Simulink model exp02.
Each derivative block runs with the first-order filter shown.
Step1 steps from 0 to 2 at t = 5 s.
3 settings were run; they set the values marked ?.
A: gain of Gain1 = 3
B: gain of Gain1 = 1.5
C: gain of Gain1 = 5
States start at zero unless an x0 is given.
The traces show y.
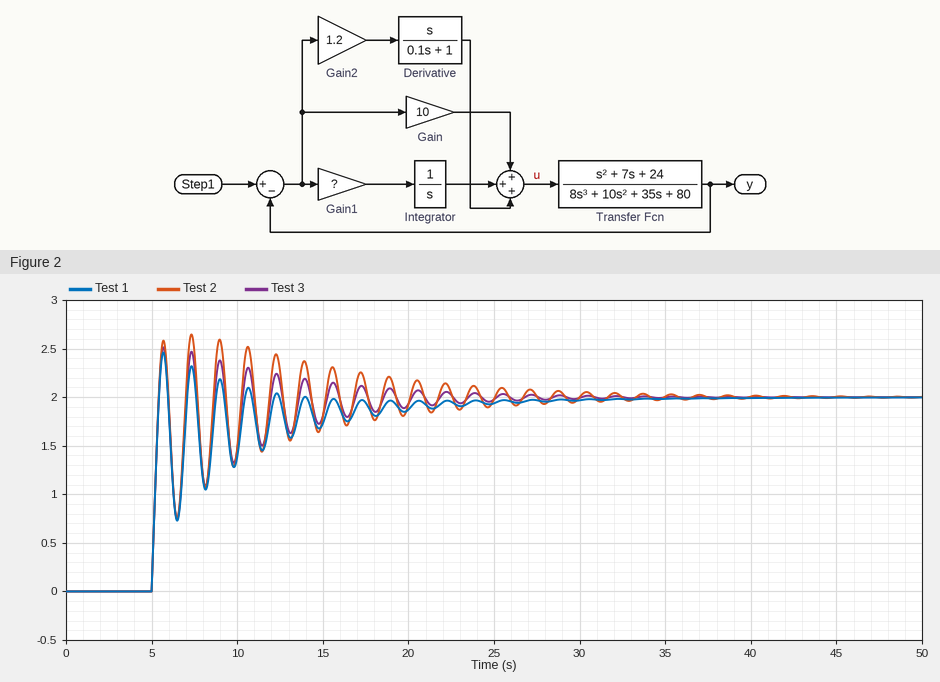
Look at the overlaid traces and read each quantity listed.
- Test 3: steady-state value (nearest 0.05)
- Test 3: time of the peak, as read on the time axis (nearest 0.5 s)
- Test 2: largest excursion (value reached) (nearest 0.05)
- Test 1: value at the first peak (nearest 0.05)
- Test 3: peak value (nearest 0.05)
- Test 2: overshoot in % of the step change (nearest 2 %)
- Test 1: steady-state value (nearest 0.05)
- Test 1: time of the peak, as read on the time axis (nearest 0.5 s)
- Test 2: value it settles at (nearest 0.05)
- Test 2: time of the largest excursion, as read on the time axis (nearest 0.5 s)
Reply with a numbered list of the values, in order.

1. 2.00
2. 5.5 s
3. 2.65
4. 2.45
5. 2.50
6. 32 %
7. 2.00
8. 5.5 s
9. 2.00
10. 7.5 s
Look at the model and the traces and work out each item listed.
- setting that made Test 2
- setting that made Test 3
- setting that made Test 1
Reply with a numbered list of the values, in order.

1. C
2. A
3. B
